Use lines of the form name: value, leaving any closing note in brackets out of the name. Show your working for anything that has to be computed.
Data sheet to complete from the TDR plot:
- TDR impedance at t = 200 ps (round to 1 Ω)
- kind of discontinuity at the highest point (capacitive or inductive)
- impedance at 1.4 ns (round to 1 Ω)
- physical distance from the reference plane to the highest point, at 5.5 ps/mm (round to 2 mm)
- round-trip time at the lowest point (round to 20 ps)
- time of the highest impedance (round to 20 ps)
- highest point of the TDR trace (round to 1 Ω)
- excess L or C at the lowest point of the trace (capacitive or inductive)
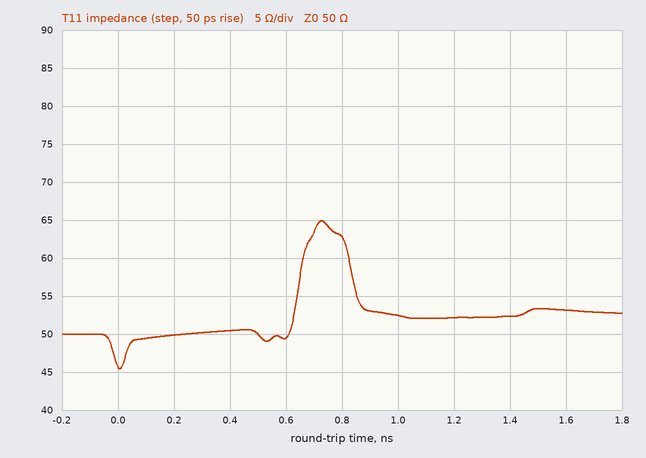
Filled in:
TDR impedance at t = 200 ps: 50 Ω
kind of discontinuity at the highest point: inductive
impedance at 1.4 ns: 52 Ω
physical distance from the reference plane to the highest point, at 5.5 ps/mm: 720 ps / 2 / 5.5 ps/mm ≈ 66 mm
round-trip time at the lowest point: 0 ps
time of the highest impedance: 720 ps
highest point of the TDR trace: 65 Ω
excess L or C at the lowest point of the trace: capacitive
